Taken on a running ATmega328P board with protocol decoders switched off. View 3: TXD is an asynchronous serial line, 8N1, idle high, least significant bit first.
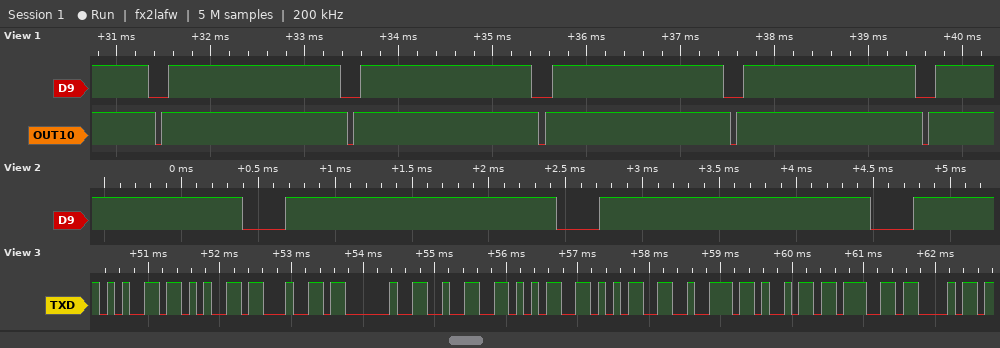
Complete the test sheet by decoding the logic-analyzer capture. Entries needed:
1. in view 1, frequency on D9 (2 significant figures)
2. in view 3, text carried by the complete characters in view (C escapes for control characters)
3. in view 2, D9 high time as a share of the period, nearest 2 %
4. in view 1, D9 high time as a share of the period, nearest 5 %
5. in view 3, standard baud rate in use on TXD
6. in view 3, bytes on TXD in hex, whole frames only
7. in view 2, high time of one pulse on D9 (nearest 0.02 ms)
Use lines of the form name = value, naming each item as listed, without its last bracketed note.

in view 1, frequency on D9 = 490 Hz
in view 3, text carried by the complete characters in view = "eed 255righ"
in view 2, D9 high time as a share of the period, nearest 2 % = 86 %
in view 1, D9 high time as a share of the period, nearest 5 % = 90 %
in view 3, standard baud rate in use on TXD = 9600 baud
in view 3, bytes on TXD in hex, whole frames only = 65 65 64 20 32 35 35 72 69 67 68
in view 2, high time of one pulse on D9 = 1.76 ms
